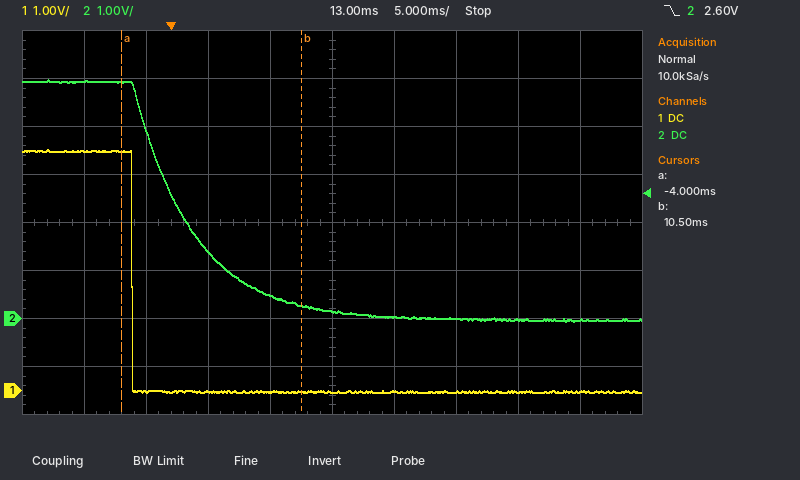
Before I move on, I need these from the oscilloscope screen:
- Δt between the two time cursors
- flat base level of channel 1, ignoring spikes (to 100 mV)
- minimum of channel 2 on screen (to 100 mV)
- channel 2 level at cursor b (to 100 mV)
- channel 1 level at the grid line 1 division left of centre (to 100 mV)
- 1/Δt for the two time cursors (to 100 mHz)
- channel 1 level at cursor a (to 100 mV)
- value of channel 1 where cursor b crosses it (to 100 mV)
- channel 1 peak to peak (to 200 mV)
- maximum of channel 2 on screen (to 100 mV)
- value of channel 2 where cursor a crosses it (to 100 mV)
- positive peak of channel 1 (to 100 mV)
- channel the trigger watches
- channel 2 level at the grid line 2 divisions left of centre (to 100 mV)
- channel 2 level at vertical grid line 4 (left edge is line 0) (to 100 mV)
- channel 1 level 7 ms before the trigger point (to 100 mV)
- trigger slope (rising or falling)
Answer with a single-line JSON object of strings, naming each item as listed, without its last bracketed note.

{"Δt between the two time cursors": "14.5 ms", "flat base level of channel 1, ignoring spikes": "0.0 V", "minimum of channel 2 on screen": "-100 mV", "channel 2 level at cursor b": "300 mV", "channel 1 level at the grid line 1 division left of centre": "0.0 V", "1/Δt for the two time cursors": "69.0 Hz", "channel 1 level at cursor a": "5.0 V", "value of channel 1 where cursor b crosses it": "0.0 V", "channel 1 peak to peak": "5.0 V", "maximum of channel 2 on screen": "5.0 V", "value of channel 2 where cursor a crosses it": "4.9 V", "positive peak of channel 1": "5.0 V", "channel the trigger watches": "channel 2", "channel 2 level at the grid line 2 divisions left of centre": "1.4 V", "channel 2 level at vertical grid line 4 (left edge is line 0)": "500 mV", "channel 1 level 7 ms before the trigger point": "5.0 V", "trigger slope": "falling"}
